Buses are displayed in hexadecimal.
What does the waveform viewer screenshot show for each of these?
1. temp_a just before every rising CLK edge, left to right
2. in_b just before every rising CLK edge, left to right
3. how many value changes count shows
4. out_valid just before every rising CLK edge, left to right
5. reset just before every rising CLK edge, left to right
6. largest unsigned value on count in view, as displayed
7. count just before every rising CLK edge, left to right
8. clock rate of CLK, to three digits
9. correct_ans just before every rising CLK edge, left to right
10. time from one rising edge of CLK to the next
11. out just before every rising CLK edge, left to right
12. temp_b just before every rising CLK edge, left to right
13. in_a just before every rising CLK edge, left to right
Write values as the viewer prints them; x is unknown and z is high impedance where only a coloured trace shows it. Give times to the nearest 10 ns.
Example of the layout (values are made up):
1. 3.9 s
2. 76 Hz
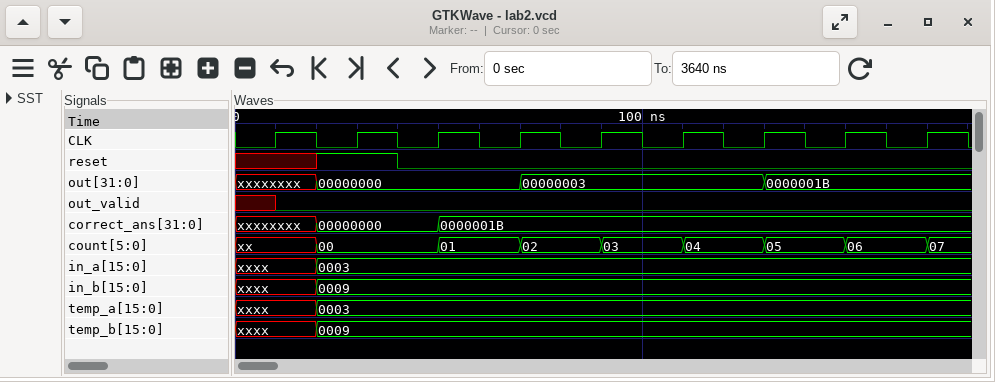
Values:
1. xxxx, 0003, 0003, 0003, 0003, 0003, 0003, 0003, 0003
2. xxxx, 0009, 0009, 0009, 0009, 0009, 0009, 0009, 0009
3. 8
4. x 0 0 0 0 0 0 0 0
5. x 1 0 0 0 0 0 0 0
6. 07
7. xx, 00, 00, 01, 02, 03, 04, 05, 06
8. 50.0 MHz
9. xxxxxxxx, 00000000, 00000000, 0000001B, 0000001B, 0000001B, 0000001B, 0000001B, 0000001B
10. 20 ns
11. xxxxxxxx, 00000000, 00000000, 00000000, 00000003, 00000003, 00000003, 0000001B, 0000001B
12. xxxx, 0009, 0009, 0009, 0009, 0009, 0009, 0009, 0009
13. xxxx, 0003, 0003, 0003, 0003, 0003, 0003, 0003, 0003
